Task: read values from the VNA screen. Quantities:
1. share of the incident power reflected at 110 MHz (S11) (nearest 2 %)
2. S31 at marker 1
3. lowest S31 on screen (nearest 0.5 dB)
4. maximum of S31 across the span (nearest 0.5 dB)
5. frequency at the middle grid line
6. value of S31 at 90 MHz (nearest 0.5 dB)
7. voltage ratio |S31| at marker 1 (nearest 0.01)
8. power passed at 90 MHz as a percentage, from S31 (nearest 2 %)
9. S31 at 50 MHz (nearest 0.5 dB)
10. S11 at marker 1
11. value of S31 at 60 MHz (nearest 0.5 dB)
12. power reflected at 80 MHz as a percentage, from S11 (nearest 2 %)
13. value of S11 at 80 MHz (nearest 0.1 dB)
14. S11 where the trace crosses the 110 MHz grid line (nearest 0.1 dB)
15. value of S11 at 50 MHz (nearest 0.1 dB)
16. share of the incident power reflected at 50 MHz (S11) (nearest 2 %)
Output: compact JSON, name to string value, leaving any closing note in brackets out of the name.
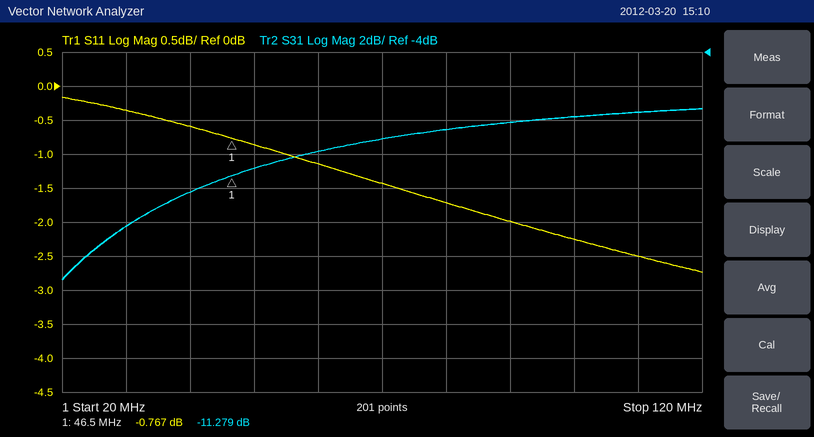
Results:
{"share of the incident power reflected at 110 MHz (S11)": "56 %", "S31 at marker 1": "-11.279 dB", "lowest S31 on screen": "-17.5 dB", "maximum of S31 across the span": "-7.5 dB", "frequency at the middle grid line": "70 MHz", "value of S31 at 90 MHz": "-8.0 dB", "voltage ratio |S31| at marker 1": "0.27", "power passed at 90 MHz as a percentage, from S31": "16 %", "S31 at 50 MHz": "-11.0 dB", "S11 at marker 1": "-0.767 dB", "value of S31 at 60 MHz": "-10.0 dB", "power reflected at 80 MHz as a percentage, from S11": "68 %", "value of S11 at 80 MHz": "-1.7 dB", "S11 where the trace crosses the 110 MHz grid line": "-2.5 dB", "value of S11 at 50 MHz": "-0.9 dB", "share of the incident power reflected at 50 MHz (S11)": "82 %"}
